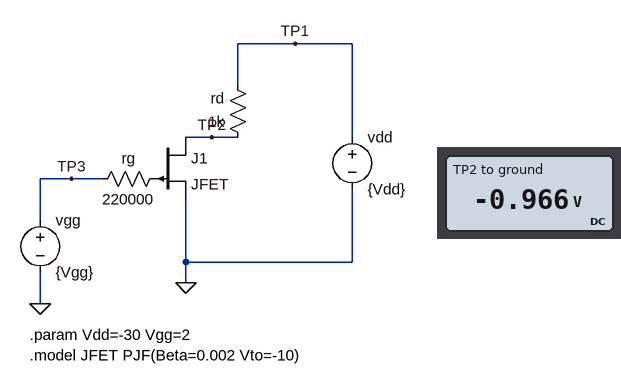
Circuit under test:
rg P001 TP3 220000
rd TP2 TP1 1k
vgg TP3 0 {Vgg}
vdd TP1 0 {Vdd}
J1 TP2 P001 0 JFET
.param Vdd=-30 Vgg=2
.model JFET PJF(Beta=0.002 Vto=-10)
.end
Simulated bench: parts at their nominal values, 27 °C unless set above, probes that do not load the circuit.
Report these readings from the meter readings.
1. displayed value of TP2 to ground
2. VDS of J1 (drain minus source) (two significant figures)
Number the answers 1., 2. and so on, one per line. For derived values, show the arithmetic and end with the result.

1. -0.966 V
2. -966 mV = -970 mV
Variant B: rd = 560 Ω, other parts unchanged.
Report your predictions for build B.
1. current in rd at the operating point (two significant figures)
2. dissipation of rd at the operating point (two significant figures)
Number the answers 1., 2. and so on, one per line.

1. 50 mA
2. 1.4 W
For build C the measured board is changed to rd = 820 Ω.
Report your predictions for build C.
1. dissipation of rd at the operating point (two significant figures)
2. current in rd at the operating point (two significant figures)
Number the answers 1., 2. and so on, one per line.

1. 1.0 W
2. 35 mA
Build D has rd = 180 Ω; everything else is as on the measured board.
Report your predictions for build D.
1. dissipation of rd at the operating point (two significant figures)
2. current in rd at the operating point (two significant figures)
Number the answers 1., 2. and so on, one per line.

1. 2.9 W
2. 130 mA
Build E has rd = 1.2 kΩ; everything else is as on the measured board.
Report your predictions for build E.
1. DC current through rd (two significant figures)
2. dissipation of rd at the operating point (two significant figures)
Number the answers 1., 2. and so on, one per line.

1. 24 mA
2. 710 mW
